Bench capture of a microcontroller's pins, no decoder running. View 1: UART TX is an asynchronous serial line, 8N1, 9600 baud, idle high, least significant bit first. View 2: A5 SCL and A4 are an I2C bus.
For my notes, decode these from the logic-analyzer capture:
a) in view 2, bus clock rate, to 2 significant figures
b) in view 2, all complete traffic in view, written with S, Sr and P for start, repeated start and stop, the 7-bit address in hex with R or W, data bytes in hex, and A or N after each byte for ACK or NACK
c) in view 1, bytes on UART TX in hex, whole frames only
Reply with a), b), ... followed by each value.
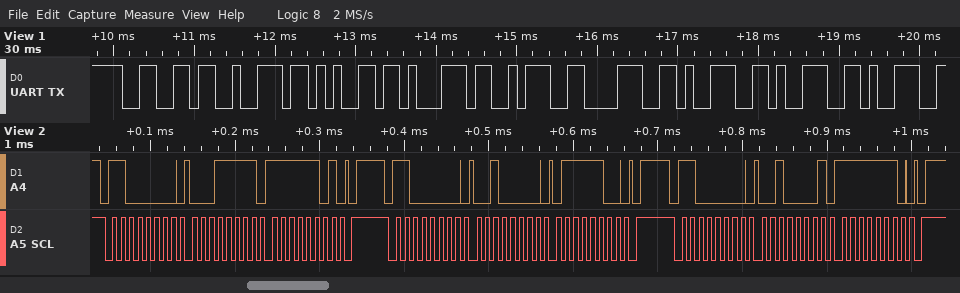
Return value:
a) 100 kHz
b) S 60W A 1F A FD A P S 60W A 20 A 7C A P S 60W A 21 A FE A P
c) 66 72 65 71 3A 38 39 39 39
